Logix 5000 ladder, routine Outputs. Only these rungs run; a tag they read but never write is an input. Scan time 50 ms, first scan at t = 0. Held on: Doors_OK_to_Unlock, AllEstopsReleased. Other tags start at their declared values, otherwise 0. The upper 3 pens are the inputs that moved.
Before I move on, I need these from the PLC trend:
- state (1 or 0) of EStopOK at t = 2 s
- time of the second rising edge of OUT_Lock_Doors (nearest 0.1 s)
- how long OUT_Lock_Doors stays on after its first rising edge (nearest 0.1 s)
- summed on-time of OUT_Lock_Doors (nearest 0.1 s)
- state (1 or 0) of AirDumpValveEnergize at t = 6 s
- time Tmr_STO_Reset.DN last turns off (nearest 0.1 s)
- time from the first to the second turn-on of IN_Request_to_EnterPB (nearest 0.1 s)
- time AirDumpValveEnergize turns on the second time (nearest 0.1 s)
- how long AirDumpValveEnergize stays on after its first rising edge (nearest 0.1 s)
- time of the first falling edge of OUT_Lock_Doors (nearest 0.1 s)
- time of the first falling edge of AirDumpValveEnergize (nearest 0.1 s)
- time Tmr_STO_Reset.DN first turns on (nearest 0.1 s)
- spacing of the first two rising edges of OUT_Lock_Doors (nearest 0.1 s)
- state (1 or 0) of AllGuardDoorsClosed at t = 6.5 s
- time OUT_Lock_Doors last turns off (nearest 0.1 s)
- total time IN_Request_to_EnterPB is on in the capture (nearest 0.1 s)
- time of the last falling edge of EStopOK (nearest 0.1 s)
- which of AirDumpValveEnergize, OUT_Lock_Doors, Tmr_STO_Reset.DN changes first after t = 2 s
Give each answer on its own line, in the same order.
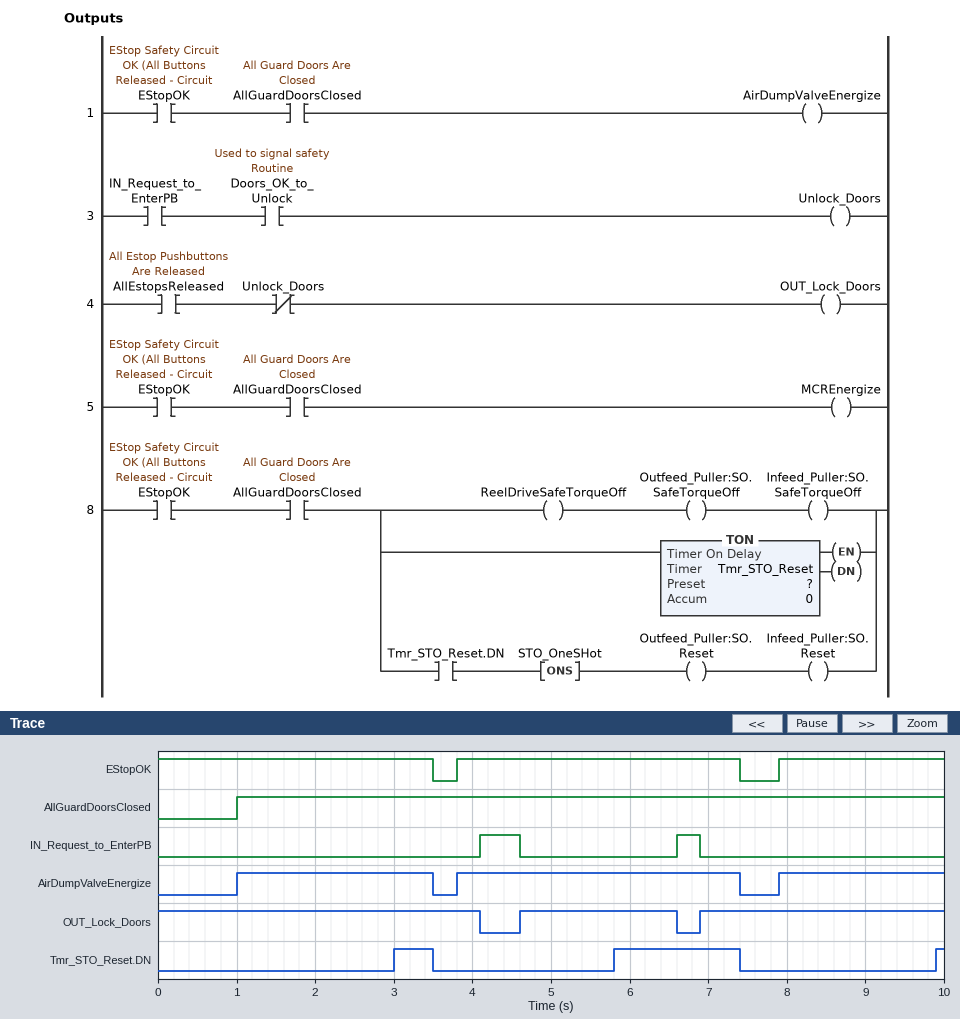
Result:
1
6.9 s
2.0 s
9.2 s
1
7.4 s
2.5 s
3.8 s
2.5 s
4.1 s
3.5 s
3.0 s
2.3 s
1
6.6 s
0.8 s
7.4 s
Tmr_STO_Reset.DN
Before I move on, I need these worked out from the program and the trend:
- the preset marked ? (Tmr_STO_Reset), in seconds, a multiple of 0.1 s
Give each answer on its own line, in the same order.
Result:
2.0 s
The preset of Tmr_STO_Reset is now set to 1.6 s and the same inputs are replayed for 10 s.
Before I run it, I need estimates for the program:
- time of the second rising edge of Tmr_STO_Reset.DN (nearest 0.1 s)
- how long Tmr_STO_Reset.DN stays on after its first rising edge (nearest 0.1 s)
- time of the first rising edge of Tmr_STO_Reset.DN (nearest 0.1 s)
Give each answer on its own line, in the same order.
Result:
5.4 s
0.9 s
2.6 s
